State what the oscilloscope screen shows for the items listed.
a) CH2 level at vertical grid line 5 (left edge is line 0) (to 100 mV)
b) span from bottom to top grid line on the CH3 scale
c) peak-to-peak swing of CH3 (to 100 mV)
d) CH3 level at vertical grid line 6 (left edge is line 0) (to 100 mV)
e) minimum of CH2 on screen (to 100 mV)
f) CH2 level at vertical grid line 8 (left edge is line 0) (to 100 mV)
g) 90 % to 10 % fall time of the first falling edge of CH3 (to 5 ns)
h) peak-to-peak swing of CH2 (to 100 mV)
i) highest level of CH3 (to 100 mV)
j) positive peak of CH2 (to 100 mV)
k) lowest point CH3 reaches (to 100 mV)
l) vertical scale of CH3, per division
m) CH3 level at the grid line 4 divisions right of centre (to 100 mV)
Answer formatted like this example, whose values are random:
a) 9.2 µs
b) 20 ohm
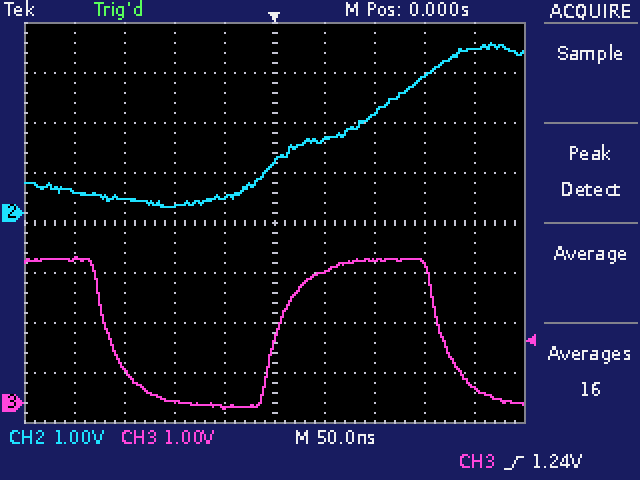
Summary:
a) 1.0 V
b) 8 V
c) 3.0 V
d) 2.6 V
e) 100 mV
f) 2.7 V
g) 50 ns
h) 3.3 V
i) 2.9 V
j) 3.4 V
k) -100 mV
l) 1 V
m) 300 mV
